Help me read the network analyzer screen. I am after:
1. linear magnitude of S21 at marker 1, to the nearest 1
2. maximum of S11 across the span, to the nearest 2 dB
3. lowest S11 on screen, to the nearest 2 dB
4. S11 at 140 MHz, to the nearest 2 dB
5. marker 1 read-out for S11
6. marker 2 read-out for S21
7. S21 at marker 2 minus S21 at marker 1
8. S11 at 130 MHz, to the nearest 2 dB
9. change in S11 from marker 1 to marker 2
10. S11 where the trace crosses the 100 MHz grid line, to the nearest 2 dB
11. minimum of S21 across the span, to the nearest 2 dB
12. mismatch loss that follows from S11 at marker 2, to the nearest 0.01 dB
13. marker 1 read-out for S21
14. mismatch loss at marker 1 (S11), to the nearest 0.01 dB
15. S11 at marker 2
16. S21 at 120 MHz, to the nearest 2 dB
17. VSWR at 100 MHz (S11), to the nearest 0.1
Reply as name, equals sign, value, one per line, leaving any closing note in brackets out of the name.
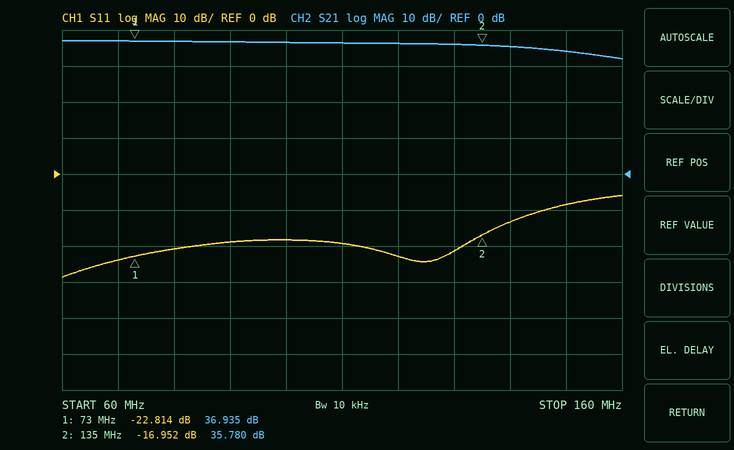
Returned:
linear magnitude of S21 at marker 1, to the nearest 1 = 70
maximum of S11 across the span, to the nearest 2 dB = -6 dB
lowest S11 on screen, to the nearest 2 dB = -28 dB
S11 at 140 MHz, to the nearest 2 dB = -14 dB
marker 1 read-out for S11 = -22.814 dB
marker 2 read-out for S21 = 35.780 dB
S21 at marker 2 minus S21 at marker 1 = -1.155 dB
S11 at 130 MHz, to the nearest 2 dB = -22 dB
change in S11 from marker 1 to marker 2 = 5.862 dB
S11 where the trace crosses the 100 MHz grid line, to the nearest 2 dB = -18 dB
minimum of S21 across the span, to the nearest 2 dB = 32 dB
mismatch loss that follows from S11 at marker 2, to the nearest 0.01 dB = 0.09 dB
marker 1 read-out for S21 = 36.935 dB
mismatch loss at marker 1 (S11), to the nearest 0.01 dB = 0.02 dB
S11 at marker 2 = -16.952 dB
S21 at 120 MHz, to the nearest 2 dB = 36 dB
VSWR at 100 MHz (S11), to the nearest 0.1 = 1.3
